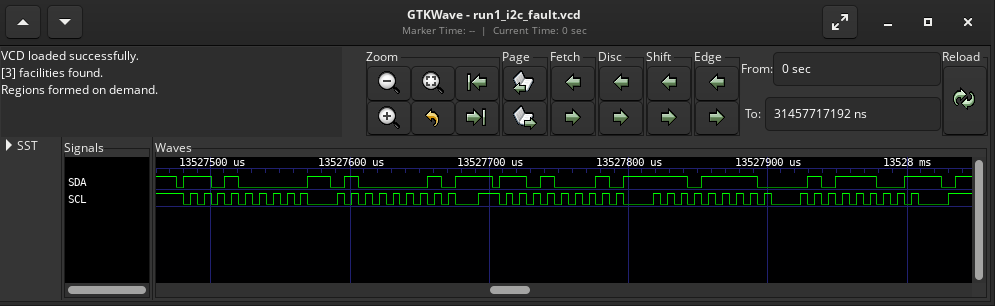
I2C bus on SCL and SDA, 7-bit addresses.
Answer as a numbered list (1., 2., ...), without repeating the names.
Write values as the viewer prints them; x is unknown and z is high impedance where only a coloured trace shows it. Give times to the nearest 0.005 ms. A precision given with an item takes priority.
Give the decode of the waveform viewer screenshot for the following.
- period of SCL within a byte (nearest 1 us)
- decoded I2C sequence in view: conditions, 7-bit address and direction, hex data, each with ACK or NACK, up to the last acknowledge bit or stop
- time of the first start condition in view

1. 10 us
2. start, address 68 write ACK, 41 ACK, repeated start, address 68 read ACK, EF ACK, 5C NACK, stop
3. 13527.475 ms
